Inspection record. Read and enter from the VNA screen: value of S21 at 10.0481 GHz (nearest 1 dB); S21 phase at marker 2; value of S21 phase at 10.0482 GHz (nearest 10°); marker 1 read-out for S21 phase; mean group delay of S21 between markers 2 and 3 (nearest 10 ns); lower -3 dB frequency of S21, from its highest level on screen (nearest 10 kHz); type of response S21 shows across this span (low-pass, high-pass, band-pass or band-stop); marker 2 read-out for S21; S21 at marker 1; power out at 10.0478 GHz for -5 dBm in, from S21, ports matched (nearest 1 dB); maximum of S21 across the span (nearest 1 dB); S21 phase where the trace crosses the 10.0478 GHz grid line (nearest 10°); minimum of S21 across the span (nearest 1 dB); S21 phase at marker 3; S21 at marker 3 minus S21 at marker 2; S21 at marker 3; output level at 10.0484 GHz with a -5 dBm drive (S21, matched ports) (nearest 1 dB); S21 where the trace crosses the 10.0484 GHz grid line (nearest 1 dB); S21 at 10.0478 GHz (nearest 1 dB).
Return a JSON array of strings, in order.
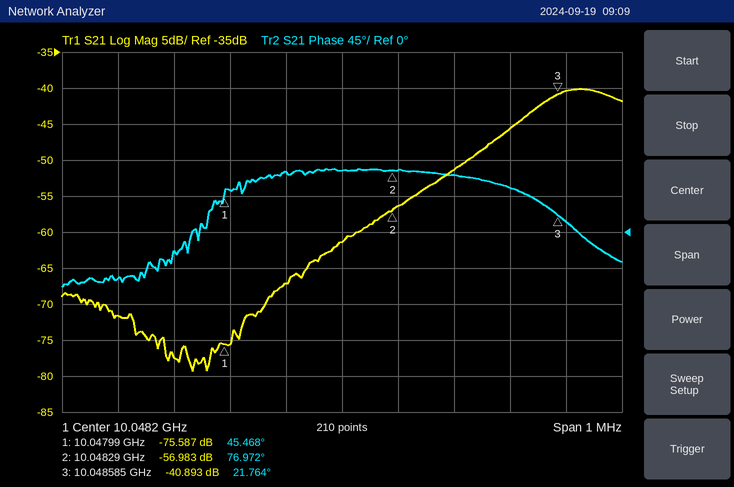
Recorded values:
["-67 dB", "76.972°", "80°", "45.468°", "520 ns", "10.04854 GHz", "high-pass", "-56.983 dB", "-75.587 dB", "-77 dBm", "-40 dB", "-60°", "-79 dB", "21.764°", "16.090 dB", "-40.893 dB", "-56 dBm", "-51 dB", "-72 dB"]
